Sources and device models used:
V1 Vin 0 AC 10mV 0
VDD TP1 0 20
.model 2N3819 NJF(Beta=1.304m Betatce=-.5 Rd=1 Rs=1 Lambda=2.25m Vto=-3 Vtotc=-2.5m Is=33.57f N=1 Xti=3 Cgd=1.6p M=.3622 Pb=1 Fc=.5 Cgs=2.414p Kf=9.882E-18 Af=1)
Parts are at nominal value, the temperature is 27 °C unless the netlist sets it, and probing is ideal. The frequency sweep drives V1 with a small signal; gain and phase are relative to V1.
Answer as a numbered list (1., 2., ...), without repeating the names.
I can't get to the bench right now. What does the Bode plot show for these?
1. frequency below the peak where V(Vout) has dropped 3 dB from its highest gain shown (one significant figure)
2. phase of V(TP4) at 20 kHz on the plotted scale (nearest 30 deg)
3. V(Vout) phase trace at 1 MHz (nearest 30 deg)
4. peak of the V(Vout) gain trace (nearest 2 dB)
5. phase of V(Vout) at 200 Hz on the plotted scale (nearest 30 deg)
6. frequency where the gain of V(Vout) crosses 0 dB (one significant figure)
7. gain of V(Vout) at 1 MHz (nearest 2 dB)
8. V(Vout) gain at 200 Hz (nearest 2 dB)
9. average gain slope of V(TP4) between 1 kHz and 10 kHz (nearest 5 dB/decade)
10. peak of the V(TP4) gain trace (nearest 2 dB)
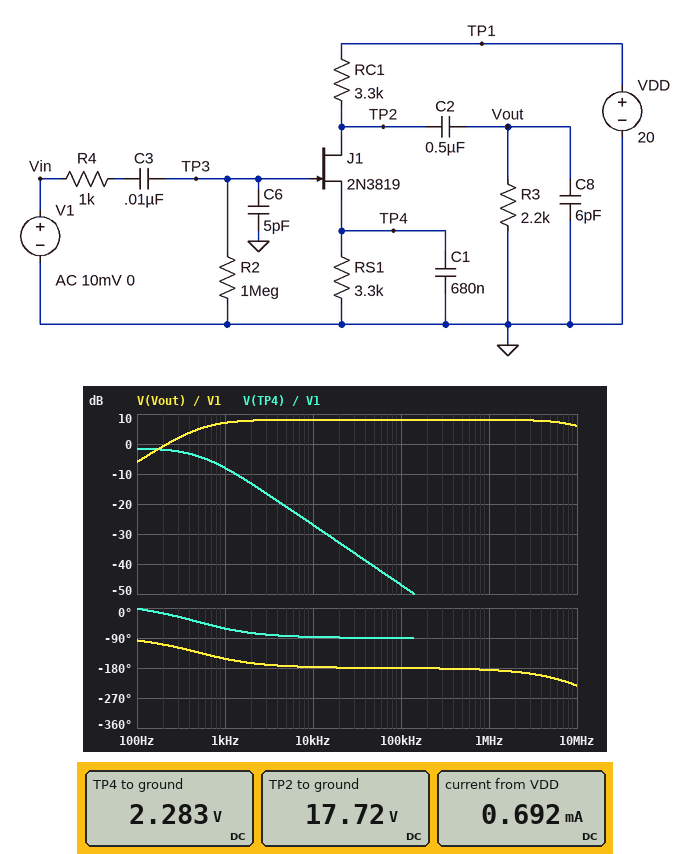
1. 500 Hz
2. -90 deg
3. -180 deg
4. 8 dB
5. -120 deg
6. 200 Hz
7. 8 dB
8. 0 dB
9. -20 dB/decade
10. -2 dB
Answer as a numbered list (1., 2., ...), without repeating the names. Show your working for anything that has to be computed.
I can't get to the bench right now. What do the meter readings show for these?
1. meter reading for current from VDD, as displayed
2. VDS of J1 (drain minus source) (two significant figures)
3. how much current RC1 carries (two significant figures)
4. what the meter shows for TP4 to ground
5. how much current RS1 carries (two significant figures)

1. 0.692 mA
2. 17.72 V - 2.283 V = 15 V
3. (20 V - 17.72 V) / 3.3 kΩ = 690 µA
4. 2.283 V
5. (2.283 V) / 3.3 kΩ = 690 µA
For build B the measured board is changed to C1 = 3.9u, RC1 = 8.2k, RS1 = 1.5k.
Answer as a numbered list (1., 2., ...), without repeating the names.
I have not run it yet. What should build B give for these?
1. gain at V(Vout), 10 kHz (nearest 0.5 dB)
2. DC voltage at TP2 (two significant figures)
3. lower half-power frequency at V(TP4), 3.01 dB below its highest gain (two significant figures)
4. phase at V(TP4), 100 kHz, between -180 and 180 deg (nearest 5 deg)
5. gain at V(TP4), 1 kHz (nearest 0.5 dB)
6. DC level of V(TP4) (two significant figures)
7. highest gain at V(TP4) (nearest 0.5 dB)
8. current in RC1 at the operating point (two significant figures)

1. 13.0 dB
2. 9.1 V
3. 13 Hz
4. -90 deg
5. -19.5 dB
6. 2.0 V
7. -3.0 dB
8. 1.3 mA
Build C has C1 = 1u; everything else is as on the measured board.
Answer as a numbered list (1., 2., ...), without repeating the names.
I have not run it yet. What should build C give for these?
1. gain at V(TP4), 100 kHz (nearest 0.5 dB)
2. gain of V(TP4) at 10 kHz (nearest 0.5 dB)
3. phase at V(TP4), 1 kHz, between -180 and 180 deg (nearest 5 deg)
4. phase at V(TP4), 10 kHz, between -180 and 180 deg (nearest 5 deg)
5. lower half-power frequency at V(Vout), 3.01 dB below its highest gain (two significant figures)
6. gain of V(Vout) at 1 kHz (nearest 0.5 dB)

1. -50.5 dB
2. -30.5 dB
3. -70 deg
4. -90 deg
5. 360 Hz
6. 7.5 dB
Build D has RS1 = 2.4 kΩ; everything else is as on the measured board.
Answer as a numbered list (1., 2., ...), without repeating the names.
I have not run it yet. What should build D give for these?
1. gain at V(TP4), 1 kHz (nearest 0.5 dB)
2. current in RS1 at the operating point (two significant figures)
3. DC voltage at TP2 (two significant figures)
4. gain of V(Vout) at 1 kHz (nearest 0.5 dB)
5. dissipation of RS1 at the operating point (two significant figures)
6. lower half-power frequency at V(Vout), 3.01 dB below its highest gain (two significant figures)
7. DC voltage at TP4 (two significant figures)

1. -7.0 dB
2. 910 µA
3. 17 V
4. 8.0 dB
5. 2.0 mW
6. 600 Hz
7. 2.2 V
